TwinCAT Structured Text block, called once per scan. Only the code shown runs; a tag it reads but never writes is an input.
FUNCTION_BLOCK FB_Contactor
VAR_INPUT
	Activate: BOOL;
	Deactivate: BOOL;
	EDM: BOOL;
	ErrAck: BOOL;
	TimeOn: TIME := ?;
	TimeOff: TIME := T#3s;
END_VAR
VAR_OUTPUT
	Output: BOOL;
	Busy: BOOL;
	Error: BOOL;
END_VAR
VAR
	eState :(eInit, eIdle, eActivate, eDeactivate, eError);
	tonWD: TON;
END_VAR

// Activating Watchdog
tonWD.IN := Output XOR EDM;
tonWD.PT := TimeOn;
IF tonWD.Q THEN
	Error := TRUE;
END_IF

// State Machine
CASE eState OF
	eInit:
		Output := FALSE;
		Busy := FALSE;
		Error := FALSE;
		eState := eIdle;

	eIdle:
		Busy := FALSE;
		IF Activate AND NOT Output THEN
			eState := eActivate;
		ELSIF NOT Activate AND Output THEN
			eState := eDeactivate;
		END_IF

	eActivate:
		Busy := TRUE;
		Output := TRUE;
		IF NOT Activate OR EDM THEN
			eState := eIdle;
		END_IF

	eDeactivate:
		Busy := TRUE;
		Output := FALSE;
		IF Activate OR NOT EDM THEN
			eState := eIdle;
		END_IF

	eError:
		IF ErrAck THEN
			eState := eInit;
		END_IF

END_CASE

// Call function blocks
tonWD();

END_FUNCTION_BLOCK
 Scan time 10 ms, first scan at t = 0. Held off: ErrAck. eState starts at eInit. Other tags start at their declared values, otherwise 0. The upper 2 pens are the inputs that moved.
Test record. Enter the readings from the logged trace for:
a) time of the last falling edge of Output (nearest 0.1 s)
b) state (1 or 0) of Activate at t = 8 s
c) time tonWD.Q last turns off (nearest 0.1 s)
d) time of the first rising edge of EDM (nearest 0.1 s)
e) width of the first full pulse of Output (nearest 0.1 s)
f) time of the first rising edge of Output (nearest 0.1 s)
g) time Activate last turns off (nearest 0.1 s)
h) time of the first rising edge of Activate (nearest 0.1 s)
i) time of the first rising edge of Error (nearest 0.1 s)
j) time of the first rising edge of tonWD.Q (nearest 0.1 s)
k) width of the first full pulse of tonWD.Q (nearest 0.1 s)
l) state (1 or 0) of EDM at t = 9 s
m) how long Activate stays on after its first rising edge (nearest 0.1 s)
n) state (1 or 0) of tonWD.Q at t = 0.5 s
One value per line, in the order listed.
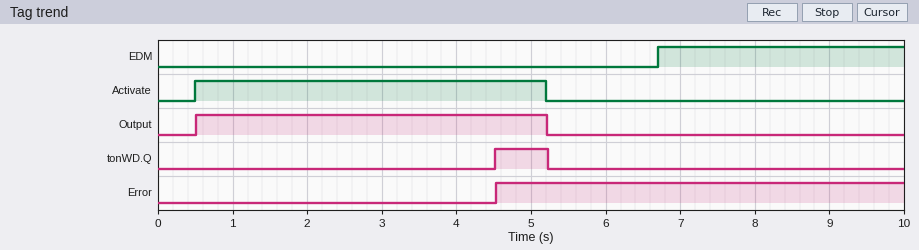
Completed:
5.2 s
0
5.2 s
6.7 s
4.7 s
0.5 s
5.2 s
0.5 s
4.5 s
4.5 s
0.7 s
1
4.7 s
0
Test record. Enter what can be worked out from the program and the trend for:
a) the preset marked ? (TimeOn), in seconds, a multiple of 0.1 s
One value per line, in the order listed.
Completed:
4.0 s
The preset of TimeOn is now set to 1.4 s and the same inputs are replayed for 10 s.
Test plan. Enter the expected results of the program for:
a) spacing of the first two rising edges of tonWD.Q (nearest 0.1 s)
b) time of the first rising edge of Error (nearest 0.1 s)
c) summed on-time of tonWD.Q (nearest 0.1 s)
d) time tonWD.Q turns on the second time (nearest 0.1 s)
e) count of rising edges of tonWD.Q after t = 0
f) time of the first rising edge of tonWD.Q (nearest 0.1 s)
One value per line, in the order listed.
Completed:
6.2 s
1.9 s
5.2 s
8.1 s
2
1.9 s
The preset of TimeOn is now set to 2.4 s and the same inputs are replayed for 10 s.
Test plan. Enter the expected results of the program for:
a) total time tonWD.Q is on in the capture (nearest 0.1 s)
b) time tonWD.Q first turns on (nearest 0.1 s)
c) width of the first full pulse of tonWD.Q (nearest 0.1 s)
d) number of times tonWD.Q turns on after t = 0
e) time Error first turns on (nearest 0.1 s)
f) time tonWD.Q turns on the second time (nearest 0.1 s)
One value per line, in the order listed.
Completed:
3.2 s
2.9 s
2.3 s
2
2.9 s
9.1 s
